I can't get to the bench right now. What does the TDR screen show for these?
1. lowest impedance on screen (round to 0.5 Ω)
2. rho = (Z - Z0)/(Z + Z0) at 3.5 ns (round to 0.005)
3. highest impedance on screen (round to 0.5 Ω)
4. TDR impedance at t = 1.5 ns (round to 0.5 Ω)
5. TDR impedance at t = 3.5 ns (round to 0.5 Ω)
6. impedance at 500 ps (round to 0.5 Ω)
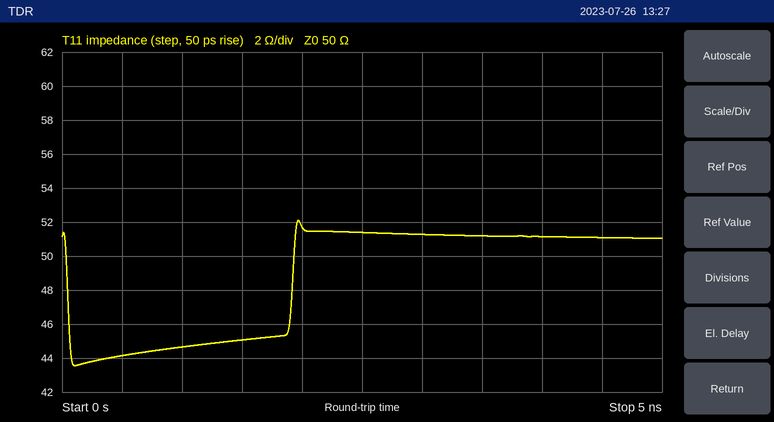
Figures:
43.5 Ω
+0.010
52.0 Ω
45.0 Ω
51.0 Ω
44.0 Ω
